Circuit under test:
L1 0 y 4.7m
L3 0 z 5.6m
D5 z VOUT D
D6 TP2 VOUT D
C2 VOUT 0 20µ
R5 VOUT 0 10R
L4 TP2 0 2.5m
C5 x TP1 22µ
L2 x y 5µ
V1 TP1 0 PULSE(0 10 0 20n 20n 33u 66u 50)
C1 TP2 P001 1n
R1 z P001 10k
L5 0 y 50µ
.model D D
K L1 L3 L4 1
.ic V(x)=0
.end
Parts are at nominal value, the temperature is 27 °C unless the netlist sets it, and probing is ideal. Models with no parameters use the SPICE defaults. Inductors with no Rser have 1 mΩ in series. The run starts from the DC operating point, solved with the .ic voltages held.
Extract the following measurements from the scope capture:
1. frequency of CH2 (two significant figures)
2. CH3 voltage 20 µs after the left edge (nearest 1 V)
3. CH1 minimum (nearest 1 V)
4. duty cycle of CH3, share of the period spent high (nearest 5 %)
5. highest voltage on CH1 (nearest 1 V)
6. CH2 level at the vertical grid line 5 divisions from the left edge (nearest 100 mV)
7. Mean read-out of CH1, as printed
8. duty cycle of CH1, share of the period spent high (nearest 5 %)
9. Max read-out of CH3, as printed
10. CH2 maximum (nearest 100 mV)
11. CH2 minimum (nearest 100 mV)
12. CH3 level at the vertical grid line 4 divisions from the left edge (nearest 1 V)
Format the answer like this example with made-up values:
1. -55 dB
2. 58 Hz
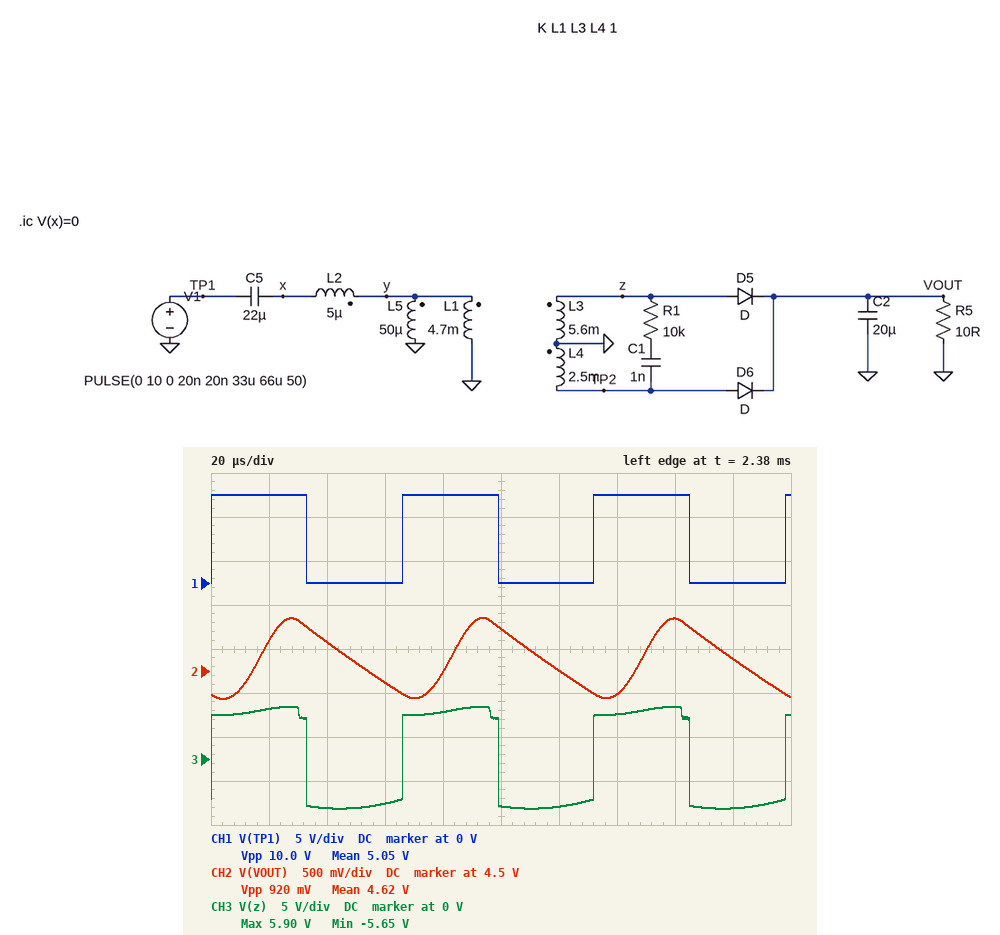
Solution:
1. 15 kHz
2. 6 V
3. 0 V
4. 50 %
5. 10 V
6. 5.0 V
7. 5.05 V
8. 50 %
9. 5.90 V
10. 5.1 V
11. 4.2 V
12. 5 V
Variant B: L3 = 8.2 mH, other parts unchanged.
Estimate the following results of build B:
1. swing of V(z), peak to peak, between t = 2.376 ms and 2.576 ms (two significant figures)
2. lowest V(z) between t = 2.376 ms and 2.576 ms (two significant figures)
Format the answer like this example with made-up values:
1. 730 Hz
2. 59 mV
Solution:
1. 14 V
2. -7.0 V
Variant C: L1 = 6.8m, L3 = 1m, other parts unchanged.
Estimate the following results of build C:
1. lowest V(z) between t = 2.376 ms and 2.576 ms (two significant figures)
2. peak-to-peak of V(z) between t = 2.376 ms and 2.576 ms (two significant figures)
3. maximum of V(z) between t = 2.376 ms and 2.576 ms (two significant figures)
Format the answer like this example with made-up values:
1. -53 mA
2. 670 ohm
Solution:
1. -2.1 V
2. 4.1 V
3. 2.0 V
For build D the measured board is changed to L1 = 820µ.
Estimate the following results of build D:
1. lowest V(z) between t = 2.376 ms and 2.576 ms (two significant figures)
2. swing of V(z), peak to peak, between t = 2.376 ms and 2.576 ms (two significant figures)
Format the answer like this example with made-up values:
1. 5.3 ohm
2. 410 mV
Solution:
1. -20 V
2. 33 V
